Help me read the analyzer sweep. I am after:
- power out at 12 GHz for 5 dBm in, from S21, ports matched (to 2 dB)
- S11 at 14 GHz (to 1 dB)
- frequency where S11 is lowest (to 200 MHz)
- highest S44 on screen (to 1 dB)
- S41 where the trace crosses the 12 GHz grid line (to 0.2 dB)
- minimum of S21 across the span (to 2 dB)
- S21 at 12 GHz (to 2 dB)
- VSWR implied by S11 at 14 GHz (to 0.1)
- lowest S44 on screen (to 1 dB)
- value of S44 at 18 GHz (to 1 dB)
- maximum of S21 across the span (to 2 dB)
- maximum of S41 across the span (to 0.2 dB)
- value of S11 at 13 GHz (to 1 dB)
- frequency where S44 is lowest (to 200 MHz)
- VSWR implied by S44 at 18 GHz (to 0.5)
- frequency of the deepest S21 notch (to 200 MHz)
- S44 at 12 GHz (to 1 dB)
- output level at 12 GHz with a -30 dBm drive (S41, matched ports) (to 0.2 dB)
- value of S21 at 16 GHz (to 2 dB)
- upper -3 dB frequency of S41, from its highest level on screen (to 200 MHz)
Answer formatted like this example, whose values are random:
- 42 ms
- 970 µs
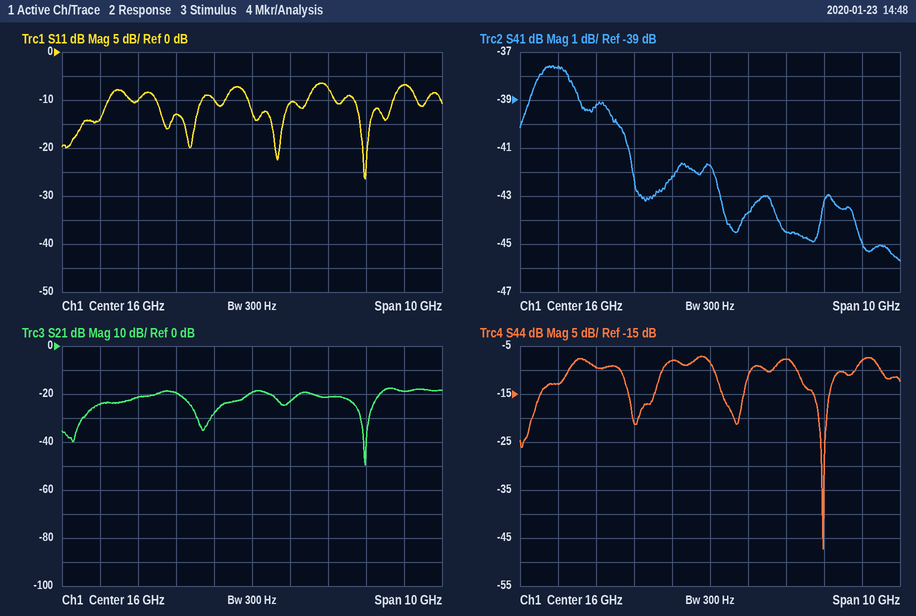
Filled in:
- -20 dBm
- -13 dB
- 19.0 GHz
- -7 dB
- -37.6 dB
- -50 dB
- -24 dB
- 1.6
- -47 dB
- -8 dB
- -18 dB
- -37.6 dB
- -10 dB
- 19.0 GHz
- 2.5
- 19.0 GHz
- -13 dB
- -67.6 dBm
- -20 dB
- 13.8 GHz
